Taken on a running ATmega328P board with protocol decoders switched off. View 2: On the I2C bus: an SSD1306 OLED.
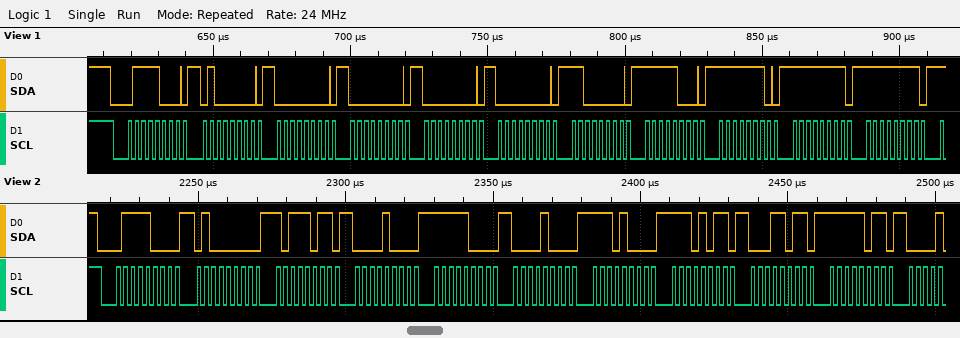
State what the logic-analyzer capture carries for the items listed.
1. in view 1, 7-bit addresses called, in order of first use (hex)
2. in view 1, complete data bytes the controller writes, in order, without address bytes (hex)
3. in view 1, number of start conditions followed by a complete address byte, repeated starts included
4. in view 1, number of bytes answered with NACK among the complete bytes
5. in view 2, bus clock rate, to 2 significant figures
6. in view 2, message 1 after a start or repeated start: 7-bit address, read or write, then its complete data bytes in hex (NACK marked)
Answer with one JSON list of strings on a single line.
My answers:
["0x3C", "40 00 00 00 00 C0 F8 FE FF FF", "1", "0", "400 kHz", "0x3C write: 40 BB 08 F8 08 E8 EB 1B FB"]
